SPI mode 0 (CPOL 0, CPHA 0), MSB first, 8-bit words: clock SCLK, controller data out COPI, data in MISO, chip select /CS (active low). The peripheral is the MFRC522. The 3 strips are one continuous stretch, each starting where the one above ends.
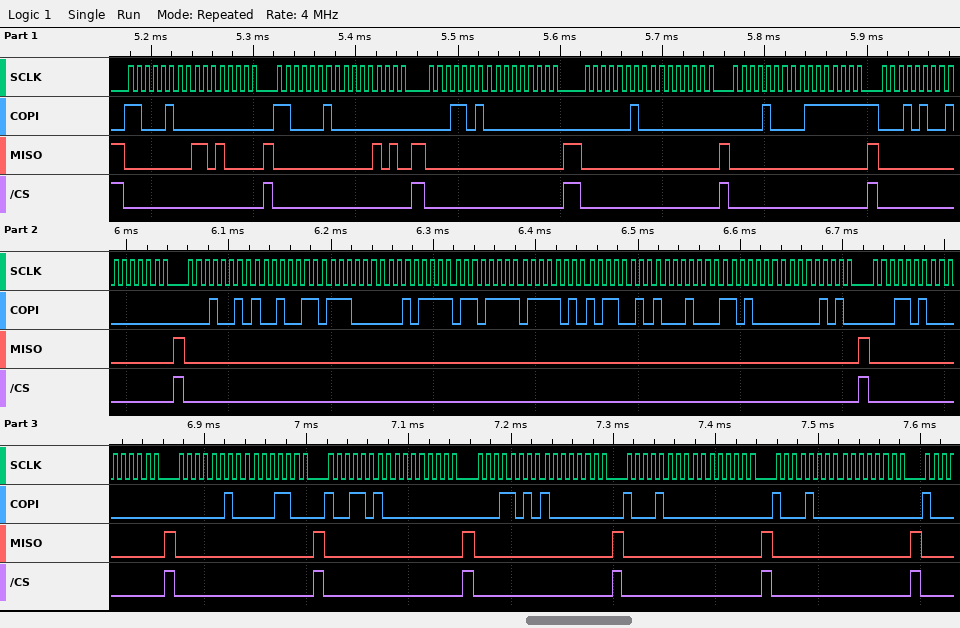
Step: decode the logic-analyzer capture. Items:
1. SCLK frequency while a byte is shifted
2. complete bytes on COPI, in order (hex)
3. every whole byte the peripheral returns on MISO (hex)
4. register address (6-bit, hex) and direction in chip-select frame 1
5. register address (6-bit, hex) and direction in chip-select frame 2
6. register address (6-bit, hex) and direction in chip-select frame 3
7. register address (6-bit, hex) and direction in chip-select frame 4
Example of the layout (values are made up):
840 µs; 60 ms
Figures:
125 kHz; C4 00 C2 00 1A 00 02 00 08 7F 14 80 12 93 70 2F 6F 7A B2 88 D0 0A 1A 00 02 0C 9A 00 1A 80 88 00 88 00; 00 D0 00 0A 00 00 00 00 00 00 00 00 00 00 00 00 00 00 00 00 00 00 00 00 00 00 00 00 00 00 00 00 00 00; 0x22 read; 0x21 read; 0x0D write; 0x01 write
